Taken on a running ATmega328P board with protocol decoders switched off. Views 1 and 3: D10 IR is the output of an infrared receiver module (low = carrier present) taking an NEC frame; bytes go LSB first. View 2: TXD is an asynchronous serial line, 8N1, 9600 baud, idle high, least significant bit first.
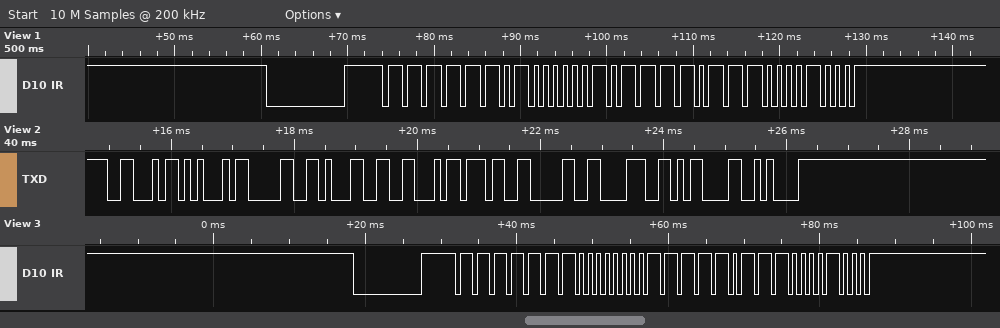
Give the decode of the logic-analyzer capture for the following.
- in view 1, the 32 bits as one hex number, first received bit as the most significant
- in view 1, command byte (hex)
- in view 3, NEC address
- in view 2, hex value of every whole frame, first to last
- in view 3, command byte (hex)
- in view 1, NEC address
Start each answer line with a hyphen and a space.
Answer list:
- 0xFD02F708
- 0xEF
- 0x7F
- 46 45 30 31 46 37 30 38 0D 0A
- 0xEF
- 0xBF
